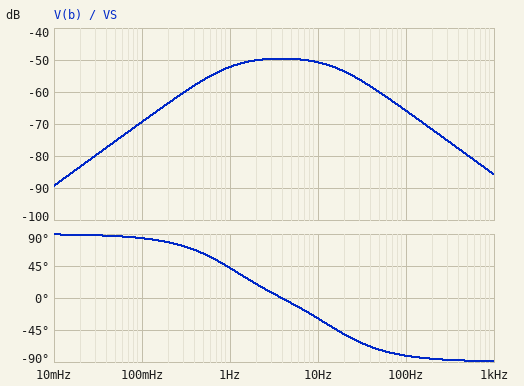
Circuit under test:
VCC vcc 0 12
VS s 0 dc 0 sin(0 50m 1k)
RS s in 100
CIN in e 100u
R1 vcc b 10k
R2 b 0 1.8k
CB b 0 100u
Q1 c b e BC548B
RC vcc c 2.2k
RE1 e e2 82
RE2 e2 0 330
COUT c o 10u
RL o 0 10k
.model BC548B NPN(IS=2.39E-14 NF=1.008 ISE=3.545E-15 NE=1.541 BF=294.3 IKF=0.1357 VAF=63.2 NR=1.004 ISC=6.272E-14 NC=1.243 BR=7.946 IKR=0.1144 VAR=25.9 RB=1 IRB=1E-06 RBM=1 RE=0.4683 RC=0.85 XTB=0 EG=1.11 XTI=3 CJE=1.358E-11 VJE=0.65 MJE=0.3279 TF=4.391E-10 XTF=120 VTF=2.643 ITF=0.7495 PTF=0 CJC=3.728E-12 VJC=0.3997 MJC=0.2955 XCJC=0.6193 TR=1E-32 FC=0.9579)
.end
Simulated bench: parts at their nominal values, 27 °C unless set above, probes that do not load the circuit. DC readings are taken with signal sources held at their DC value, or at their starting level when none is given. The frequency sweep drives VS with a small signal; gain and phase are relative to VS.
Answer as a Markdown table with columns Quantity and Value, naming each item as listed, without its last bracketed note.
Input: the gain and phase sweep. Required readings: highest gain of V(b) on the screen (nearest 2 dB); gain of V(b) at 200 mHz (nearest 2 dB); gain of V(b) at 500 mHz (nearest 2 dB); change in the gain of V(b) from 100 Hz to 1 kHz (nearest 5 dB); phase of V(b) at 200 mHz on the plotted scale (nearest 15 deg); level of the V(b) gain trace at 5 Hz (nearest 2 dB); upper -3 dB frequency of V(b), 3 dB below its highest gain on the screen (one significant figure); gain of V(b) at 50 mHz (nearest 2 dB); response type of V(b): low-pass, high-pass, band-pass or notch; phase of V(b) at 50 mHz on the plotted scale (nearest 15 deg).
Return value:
| Quantity | Value |
|---|---|
| highest gain of V(b) on the screen | -50 dB |
| gain of V(b) at 200 mHz | -64 dB |
| gain of V(b) at 500 mHz | -56 dB |
| change in the gain of V(b) from 100 Hz to 1 kHz | -20 dB |
| phase of V(b) at 200 mHz on the plotted scale | 75 deg |
| level of the V(b) gain trace at 5 Hz | -50 dB |
| upper -3 dB frequency of V(b), 3 dB below its highest gain on the screen | 20 Hz |
| gain of V(b) at 50 mHz | -76 dB |
| response type of V(b): low-pass, high-pass, band-pass or notch | band-pass |
| phase of V(b) at 50 mHz on the plotted scale | 90 deg |
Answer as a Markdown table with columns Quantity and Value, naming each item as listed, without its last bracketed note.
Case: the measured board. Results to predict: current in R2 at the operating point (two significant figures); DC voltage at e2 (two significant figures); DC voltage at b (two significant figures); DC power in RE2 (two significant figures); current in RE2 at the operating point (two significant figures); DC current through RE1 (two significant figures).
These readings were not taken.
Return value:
| Quantity | Value |
|---|---|
| current in R2 at the operating point | 1.0 mA |
| DC voltage at e2 | 920 mV |
| DC voltage at b | 1.8 V |
| DC power in RE2 | 2.6 mW |
| current in RE2 at the operating point | 2.8 mA |
| DC current through RE1 | 2.8 mA |
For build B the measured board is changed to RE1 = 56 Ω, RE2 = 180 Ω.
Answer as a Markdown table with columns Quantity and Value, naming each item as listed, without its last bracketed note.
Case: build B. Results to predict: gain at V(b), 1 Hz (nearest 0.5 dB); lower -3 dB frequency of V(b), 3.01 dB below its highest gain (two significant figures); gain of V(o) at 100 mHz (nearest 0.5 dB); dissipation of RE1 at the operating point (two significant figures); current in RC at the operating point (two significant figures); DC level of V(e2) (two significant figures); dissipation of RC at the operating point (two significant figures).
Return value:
| Quantity | Value |
|---|---|
| gain at V(b), 1 Hz | -51.0 dB |
| lower -3 dB frequency of V(b), 3.01 dB below its highest gain | 920 mHz |
| gain of V(o) at 100 mHz | -42.0 dB |
| dissipation of RE1 at the operating point | 1.3 mW |
| current in RC at the operating point | 4.7 mA |
| DC level of V(e2) | 860 mV |
| dissipation of RC at the operating point | 49 mW |
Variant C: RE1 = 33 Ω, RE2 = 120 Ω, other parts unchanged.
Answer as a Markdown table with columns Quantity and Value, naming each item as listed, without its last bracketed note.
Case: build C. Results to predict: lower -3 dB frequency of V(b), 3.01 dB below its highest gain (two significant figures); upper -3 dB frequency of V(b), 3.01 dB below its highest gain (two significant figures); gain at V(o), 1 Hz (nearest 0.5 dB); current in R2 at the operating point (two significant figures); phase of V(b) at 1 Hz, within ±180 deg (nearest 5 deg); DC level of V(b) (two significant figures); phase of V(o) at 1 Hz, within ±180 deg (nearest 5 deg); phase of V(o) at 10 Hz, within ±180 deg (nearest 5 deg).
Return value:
| Quantity | Value |
|---|---|
| lower -3 dB frequency of V(b), 3.01 dB below its highest gain | 3.6 Hz |
| upper -3 dB frequency of V(b), 3.01 dB below its highest gain | 34 Hz |
| gain at V(o), 1 Hz | -27.0 dB |
| current in R2 at the operating point | 830 µA |
| phase of V(b) at 1 Hz, within ±180 deg | 75 deg |
| DC level of V(b) | 1.5 V |
| phase of V(o) at 1 Hz, within ±180 deg | 140 deg |
| phase of V(o) at 10 Hz, within ±180 deg | 50 deg |
